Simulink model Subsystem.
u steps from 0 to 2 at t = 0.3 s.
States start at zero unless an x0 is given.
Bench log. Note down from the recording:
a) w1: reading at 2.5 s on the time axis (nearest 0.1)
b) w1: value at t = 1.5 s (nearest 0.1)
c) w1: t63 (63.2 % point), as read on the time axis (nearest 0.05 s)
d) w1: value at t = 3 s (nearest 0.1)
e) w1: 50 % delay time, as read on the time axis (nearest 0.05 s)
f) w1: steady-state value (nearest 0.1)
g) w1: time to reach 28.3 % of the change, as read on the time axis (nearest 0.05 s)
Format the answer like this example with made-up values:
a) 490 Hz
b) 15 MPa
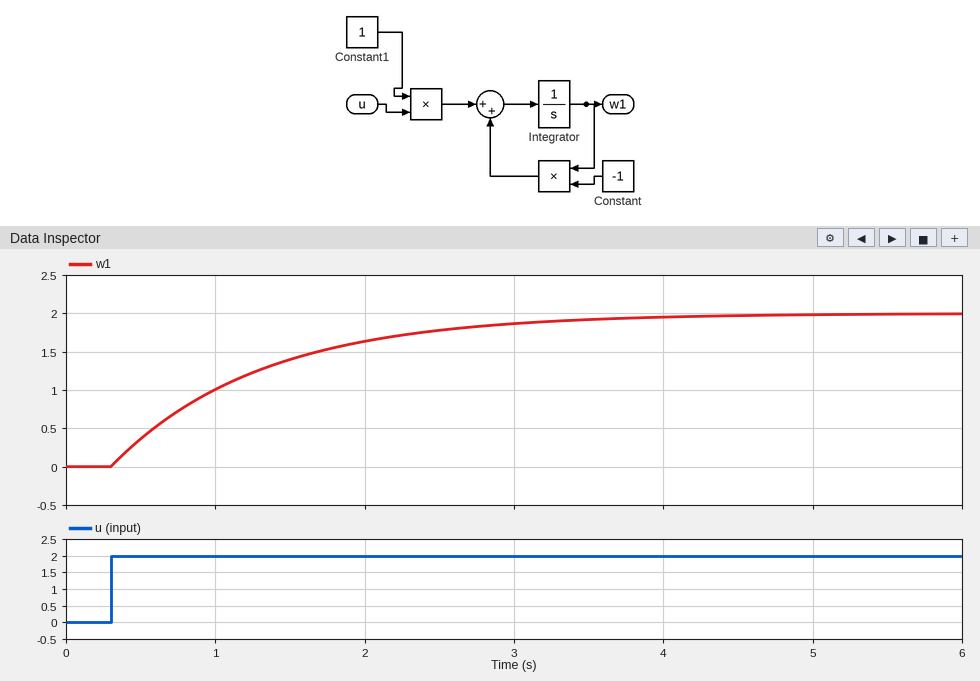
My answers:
a) 1.8
b) 1.4
c) 1.30 s
d) 1.9
e) 1.00 s
f) 2.0
g) 0.65 s
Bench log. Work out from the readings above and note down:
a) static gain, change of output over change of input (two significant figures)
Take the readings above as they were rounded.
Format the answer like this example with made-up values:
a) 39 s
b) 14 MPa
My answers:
a) 1.0
